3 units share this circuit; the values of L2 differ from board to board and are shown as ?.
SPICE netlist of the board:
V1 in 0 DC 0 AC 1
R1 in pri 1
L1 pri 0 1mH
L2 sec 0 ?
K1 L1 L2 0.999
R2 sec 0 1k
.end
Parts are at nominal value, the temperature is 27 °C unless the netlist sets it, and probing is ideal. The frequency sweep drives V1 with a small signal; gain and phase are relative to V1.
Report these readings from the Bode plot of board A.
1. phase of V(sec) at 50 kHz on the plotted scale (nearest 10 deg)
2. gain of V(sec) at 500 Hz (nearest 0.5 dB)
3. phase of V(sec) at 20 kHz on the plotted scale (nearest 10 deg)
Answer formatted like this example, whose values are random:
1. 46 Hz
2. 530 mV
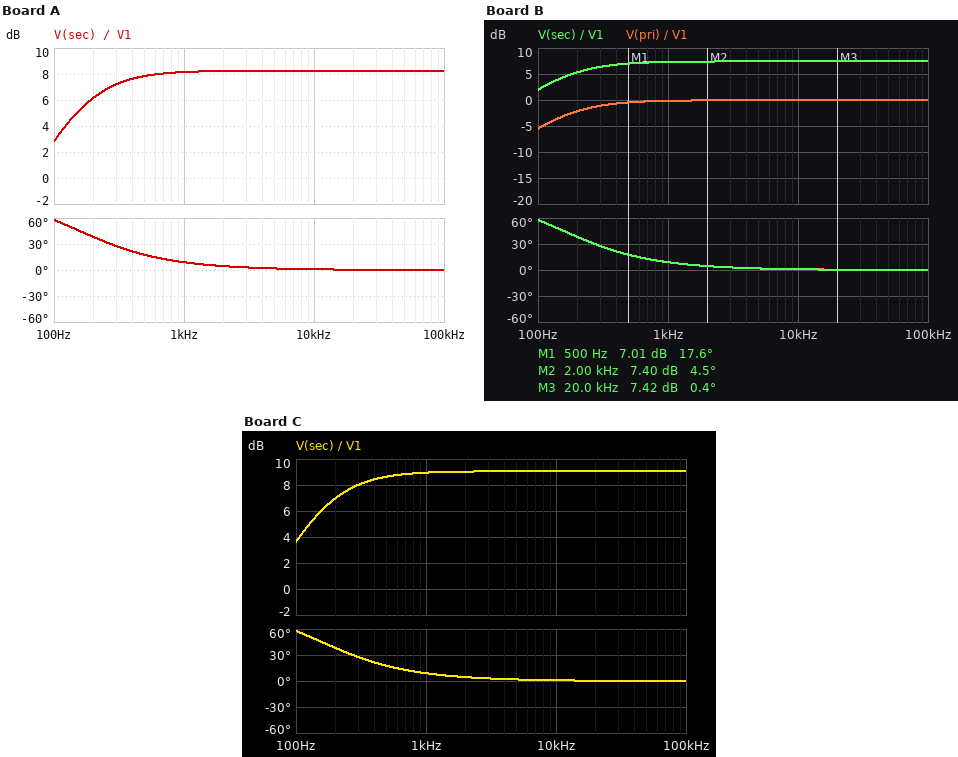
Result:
1. 0 deg
2. 8.0 dB
3. 0 deg
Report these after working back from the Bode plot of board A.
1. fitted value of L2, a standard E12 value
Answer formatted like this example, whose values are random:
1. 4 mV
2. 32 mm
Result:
1. 6.8 mH
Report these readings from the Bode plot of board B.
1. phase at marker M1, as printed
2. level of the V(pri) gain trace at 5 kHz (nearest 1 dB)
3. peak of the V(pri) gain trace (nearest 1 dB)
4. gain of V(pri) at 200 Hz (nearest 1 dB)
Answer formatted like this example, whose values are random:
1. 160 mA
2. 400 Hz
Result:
1. 17.6 deg
2. 0 dB
3. 0 dB
4. -2 dB
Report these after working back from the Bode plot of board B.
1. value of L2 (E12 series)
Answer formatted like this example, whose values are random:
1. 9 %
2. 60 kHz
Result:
1. 5.6 mH
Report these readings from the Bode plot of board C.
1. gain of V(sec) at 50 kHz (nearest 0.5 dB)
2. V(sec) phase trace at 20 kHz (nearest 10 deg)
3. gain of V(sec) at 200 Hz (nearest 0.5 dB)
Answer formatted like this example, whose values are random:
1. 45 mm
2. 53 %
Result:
1. 9.0 dB
2. 0 deg
3. 7.0 dB
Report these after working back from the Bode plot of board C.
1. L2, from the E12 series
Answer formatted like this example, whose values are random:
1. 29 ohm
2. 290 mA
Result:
1. 8.2 mH
